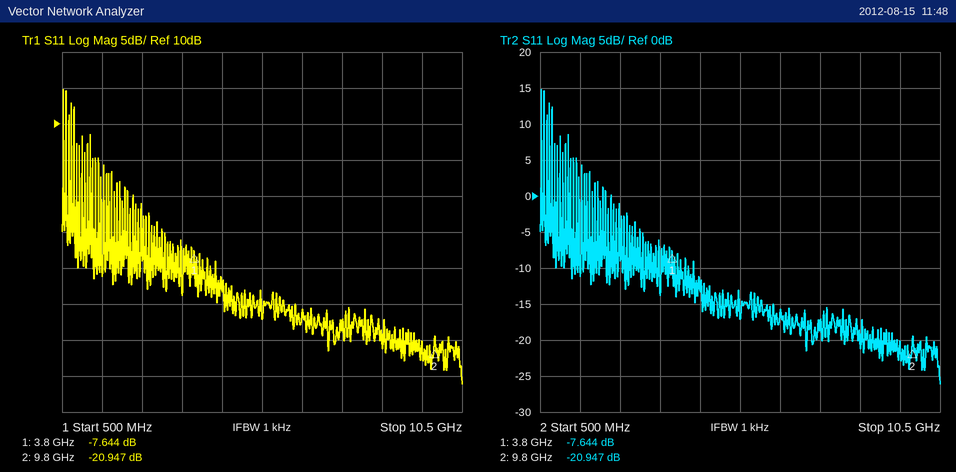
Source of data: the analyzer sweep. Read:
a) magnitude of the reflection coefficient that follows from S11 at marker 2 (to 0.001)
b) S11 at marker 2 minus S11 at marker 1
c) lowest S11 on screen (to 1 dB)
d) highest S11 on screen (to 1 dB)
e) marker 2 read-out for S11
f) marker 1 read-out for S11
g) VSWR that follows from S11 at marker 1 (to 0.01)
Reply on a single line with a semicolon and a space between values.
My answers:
0.090; -13.303 dB; -26 dB; 15 dB; -20.947 dB; -7.644 dB; 2.42
